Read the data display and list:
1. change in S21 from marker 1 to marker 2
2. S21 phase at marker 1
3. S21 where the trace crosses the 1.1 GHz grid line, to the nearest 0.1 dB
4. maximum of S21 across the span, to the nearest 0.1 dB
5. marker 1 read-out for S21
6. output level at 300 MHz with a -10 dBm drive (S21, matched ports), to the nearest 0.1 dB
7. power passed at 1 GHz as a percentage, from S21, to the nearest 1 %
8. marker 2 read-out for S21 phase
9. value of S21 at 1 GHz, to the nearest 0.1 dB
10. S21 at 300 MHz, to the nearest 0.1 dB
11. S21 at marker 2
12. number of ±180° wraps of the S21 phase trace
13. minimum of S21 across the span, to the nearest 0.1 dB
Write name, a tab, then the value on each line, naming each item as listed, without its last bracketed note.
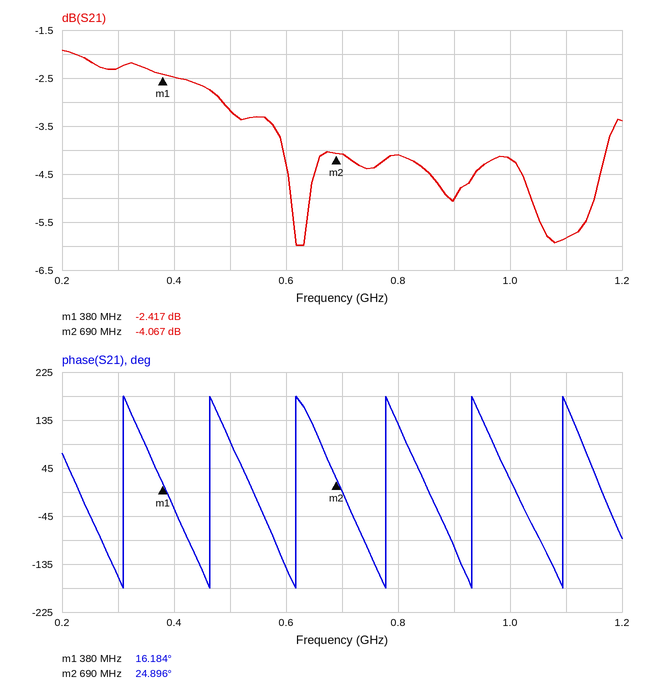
change in S21 from marker 1 to marker 2	-1.650 dB
S21 phase at marker 1	16.184°
S21 where the trace crosses the 1.1 GHz grid line, to the nearest 0.1 dB	-5.8 dB
maximum of S21 across the span, to the nearest 0.1 dB	-1.9 dB
marker 1 read-out for S21	-2.417 dB
output level at 300 MHz with a -10 dBm drive (S21, matched ports), to the nearest 0.1 dB	-12.3 dBm
power passed at 1 GHz as a percentage, from S21, to the nearest 1 %	38 %
marker 2 read-out for S21 phase	24.896°
value of S21 at 1 GHz, to the nearest 0.1 dB	-4.2 dB
S21 at 300 MHz, to the nearest 0.1 dB	-2.3 dB
S21 at marker 2	-4.067 dB
number of ±180° wraps of the S21 phase trace	6
minimum of S21 across the span, to the nearest 0.1 dB	-6.0 dB
